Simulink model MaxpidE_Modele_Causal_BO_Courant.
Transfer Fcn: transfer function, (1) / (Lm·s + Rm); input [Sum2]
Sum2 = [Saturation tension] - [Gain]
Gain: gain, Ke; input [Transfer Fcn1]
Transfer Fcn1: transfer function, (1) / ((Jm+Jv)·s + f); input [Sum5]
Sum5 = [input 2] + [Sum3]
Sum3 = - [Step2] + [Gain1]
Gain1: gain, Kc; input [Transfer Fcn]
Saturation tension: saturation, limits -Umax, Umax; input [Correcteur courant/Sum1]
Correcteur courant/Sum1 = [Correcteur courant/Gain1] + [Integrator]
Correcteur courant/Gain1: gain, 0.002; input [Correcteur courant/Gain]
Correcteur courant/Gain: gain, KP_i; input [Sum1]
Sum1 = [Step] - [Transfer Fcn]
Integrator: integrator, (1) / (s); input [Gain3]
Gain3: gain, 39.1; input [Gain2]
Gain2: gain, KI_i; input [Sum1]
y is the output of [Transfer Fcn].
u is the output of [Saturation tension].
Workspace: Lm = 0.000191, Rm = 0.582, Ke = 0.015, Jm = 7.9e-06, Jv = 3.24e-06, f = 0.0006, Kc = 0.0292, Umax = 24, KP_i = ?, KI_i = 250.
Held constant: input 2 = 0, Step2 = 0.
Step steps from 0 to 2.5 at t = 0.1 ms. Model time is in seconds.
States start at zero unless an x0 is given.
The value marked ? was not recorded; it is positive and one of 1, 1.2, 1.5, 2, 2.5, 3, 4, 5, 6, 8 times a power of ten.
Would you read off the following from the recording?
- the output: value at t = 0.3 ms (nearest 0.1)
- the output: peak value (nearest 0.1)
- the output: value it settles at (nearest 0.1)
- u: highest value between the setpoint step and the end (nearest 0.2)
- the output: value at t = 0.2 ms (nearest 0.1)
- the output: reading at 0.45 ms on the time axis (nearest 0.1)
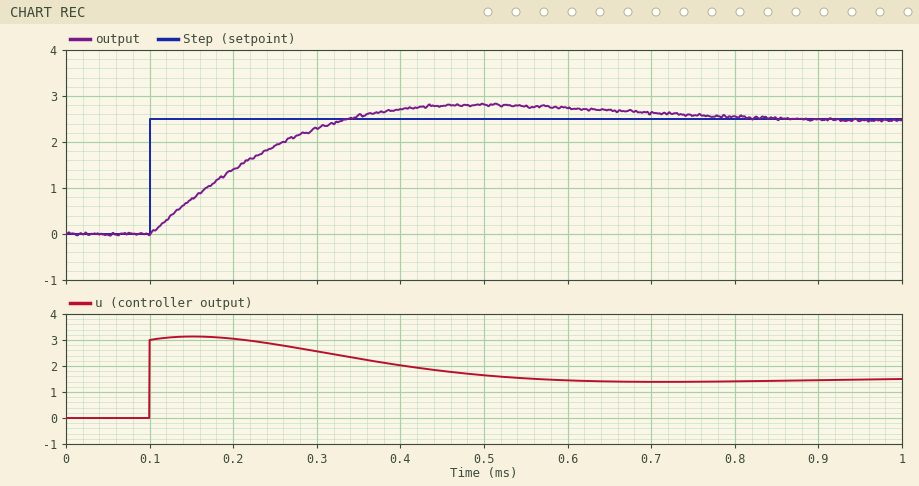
2.3
2.8
2.5
3.2
1.4
2.8
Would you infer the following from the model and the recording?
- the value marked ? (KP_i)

600
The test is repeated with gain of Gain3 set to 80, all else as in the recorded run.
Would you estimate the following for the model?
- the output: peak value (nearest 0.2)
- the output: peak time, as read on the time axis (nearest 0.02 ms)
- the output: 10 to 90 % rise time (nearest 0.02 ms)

3.2
0.38 ms
0.12 ms
